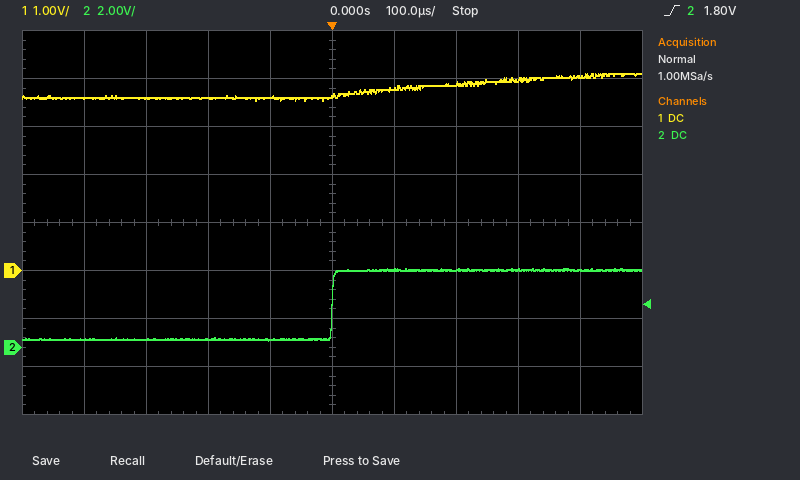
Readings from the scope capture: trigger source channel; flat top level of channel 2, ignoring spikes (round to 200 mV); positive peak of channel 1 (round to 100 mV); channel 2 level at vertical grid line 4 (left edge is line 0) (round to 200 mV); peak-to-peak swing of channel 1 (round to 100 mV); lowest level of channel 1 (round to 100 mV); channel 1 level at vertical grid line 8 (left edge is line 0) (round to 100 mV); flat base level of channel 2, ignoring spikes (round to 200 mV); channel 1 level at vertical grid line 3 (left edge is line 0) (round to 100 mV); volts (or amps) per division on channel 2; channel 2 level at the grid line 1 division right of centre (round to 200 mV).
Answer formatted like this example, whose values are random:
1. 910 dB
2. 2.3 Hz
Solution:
1. channel 2
2. 3.2 V
3. 4.1 V
4. 400 mV
5. 600 mV
6. 3.5 V
7. 4.0 V
8. 400 mV
9. 3.6 V
10. 2 V
11. 3.2 V
